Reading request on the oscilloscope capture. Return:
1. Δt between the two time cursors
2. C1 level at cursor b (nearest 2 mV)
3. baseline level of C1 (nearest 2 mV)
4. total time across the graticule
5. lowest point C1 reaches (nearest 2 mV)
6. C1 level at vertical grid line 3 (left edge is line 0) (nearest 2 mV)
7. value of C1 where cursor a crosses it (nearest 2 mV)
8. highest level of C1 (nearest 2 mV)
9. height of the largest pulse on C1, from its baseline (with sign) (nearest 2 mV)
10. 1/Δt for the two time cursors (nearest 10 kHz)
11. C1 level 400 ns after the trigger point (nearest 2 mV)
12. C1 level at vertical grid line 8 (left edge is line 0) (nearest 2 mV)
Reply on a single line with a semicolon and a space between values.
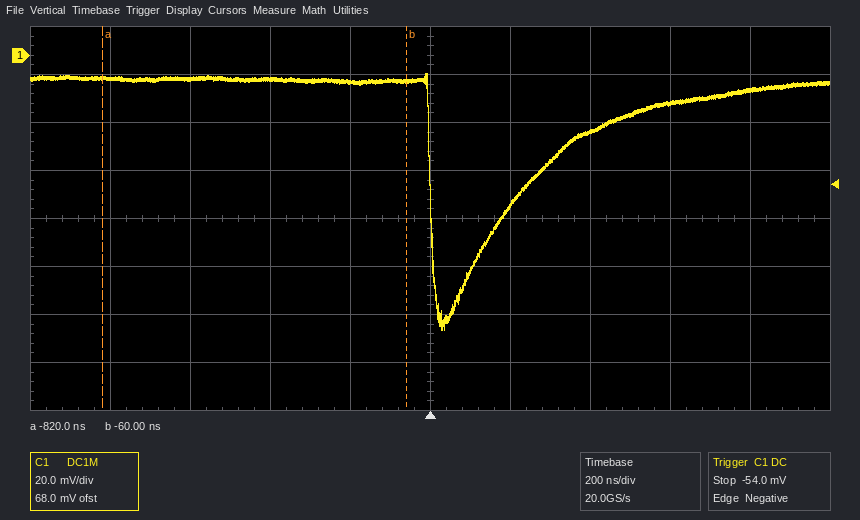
760 ns; -10 mV; -10 mV; 2 µs; -114 mV; -10 mV; -10 mV; -8 mV; -104 mV; 1.32 MHz; -32 mV; -20 mV
